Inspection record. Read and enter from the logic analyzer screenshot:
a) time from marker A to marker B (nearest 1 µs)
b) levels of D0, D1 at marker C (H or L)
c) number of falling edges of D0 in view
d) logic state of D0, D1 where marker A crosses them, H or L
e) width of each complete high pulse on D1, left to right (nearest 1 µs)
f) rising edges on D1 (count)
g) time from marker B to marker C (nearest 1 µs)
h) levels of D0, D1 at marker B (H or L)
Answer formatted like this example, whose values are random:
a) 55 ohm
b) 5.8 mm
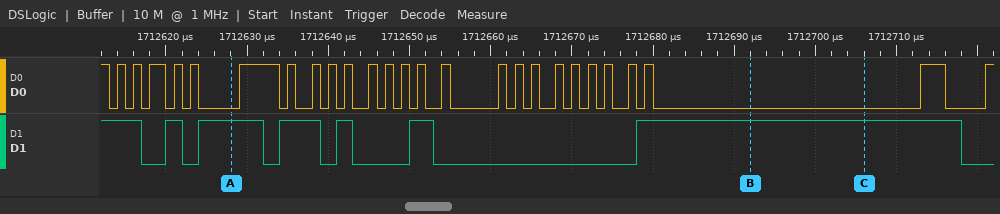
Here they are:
a) 64 µs
b) D0=L, D1=H
c) 26
d) D0=L, D1=H
e) 2 µs, 8 µs, 5 µs, 2 µs, 3 µs, 40 µs
f) 6
g) 14 µs
h) D0=L, D1=H
